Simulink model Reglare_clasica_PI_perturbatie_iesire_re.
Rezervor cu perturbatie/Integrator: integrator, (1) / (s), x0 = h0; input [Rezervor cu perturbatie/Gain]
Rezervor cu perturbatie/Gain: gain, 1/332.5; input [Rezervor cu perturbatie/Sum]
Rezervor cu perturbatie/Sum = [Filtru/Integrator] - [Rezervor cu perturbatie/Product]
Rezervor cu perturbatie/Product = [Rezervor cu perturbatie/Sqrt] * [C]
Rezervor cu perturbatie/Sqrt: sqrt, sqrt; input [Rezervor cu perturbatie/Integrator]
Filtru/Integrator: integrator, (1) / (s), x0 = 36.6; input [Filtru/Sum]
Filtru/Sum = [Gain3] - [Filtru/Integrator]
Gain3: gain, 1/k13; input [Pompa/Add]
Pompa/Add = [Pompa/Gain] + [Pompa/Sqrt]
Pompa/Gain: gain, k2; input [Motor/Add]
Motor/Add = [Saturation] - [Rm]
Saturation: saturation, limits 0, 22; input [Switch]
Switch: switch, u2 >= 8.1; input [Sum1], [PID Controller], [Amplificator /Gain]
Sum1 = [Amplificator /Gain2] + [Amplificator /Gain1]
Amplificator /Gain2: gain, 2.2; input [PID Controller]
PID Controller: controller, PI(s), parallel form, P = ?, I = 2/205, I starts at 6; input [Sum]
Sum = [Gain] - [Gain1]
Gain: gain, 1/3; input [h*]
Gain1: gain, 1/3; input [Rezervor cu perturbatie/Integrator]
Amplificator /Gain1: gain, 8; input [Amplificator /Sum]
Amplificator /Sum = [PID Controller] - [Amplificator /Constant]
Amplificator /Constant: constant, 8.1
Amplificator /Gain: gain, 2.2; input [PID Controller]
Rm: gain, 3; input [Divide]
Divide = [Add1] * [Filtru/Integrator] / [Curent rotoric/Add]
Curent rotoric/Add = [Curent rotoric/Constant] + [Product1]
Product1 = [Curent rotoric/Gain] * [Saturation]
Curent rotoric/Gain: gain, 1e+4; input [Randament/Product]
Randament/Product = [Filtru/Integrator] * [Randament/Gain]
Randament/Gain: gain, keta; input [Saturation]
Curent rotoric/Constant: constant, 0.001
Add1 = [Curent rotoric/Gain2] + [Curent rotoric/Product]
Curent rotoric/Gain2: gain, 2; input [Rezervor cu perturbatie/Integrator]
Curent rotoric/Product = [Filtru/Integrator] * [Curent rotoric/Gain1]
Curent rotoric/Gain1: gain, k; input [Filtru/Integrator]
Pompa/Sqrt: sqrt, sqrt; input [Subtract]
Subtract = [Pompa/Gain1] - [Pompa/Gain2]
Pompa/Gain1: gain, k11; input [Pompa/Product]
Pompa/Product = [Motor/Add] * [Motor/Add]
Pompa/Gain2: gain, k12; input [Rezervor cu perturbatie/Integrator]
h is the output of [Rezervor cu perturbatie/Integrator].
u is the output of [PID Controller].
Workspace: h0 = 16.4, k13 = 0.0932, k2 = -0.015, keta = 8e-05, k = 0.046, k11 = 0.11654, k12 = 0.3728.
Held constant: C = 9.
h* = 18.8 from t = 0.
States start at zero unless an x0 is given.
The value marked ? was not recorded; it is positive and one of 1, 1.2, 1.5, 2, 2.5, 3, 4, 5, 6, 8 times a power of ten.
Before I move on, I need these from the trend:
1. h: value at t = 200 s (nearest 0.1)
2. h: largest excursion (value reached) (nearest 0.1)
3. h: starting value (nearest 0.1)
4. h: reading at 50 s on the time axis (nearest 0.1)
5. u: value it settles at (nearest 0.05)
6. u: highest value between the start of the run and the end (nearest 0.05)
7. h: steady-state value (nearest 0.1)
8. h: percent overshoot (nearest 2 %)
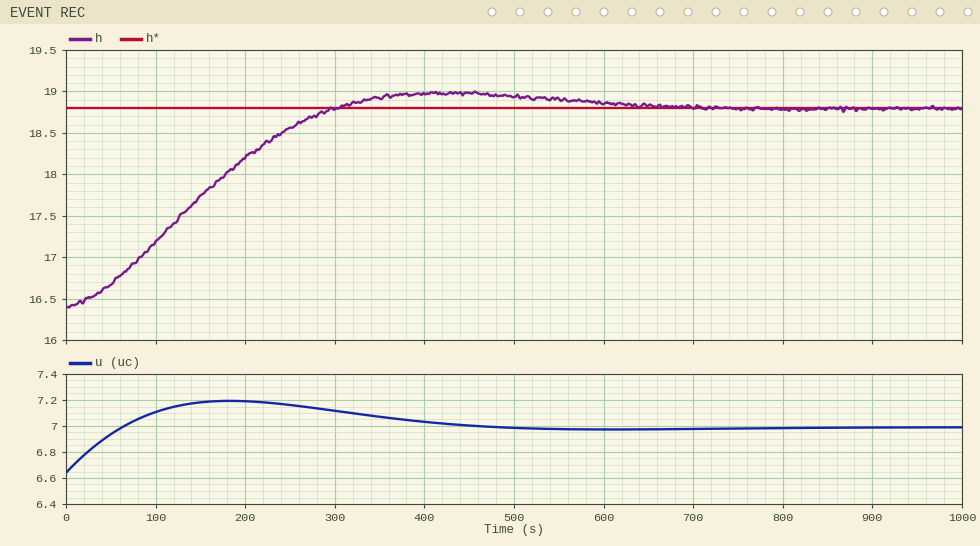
18.2
19.0
16.4
16.7
7.00
7.20
18.8
8 %
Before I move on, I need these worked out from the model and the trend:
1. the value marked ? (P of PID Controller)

0.8
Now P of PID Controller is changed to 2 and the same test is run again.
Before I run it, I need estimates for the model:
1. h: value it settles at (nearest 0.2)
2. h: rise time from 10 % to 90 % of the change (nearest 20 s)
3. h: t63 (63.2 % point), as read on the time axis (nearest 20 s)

18.8
320 s
100 s
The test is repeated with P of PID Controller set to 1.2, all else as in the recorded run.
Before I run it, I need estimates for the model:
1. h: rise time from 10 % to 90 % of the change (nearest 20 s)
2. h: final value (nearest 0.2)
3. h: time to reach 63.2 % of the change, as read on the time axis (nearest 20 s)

240 s
18.8
140 s
